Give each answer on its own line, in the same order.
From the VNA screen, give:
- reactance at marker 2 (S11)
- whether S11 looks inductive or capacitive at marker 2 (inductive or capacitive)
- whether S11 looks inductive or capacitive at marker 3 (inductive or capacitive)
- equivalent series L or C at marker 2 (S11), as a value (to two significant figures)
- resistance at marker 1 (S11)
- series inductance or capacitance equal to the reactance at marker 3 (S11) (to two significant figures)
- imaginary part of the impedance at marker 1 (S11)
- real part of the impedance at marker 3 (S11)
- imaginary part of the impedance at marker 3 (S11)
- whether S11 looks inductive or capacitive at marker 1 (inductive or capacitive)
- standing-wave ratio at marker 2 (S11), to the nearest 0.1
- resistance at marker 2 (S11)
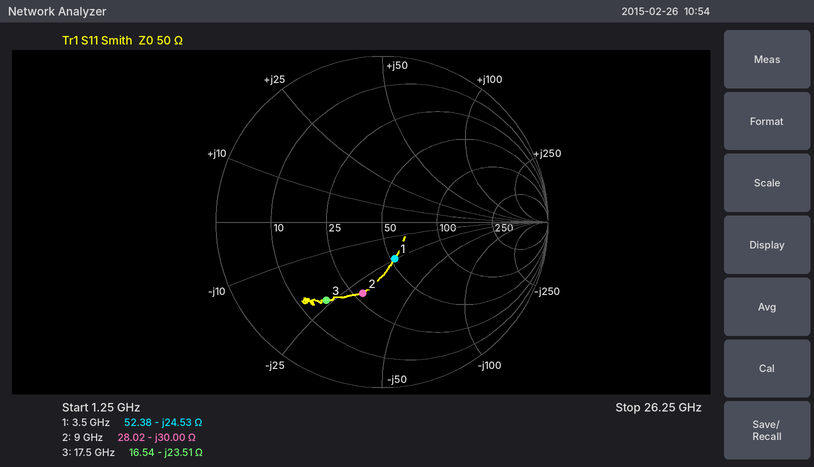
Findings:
-30.00 Ω
capacitive
capacitive
590 fF
52.38 Ω
390 fF
-24.53 Ω
16.54 Ω
-23.51 Ω
capacitive
2.6
28.02 Ω
